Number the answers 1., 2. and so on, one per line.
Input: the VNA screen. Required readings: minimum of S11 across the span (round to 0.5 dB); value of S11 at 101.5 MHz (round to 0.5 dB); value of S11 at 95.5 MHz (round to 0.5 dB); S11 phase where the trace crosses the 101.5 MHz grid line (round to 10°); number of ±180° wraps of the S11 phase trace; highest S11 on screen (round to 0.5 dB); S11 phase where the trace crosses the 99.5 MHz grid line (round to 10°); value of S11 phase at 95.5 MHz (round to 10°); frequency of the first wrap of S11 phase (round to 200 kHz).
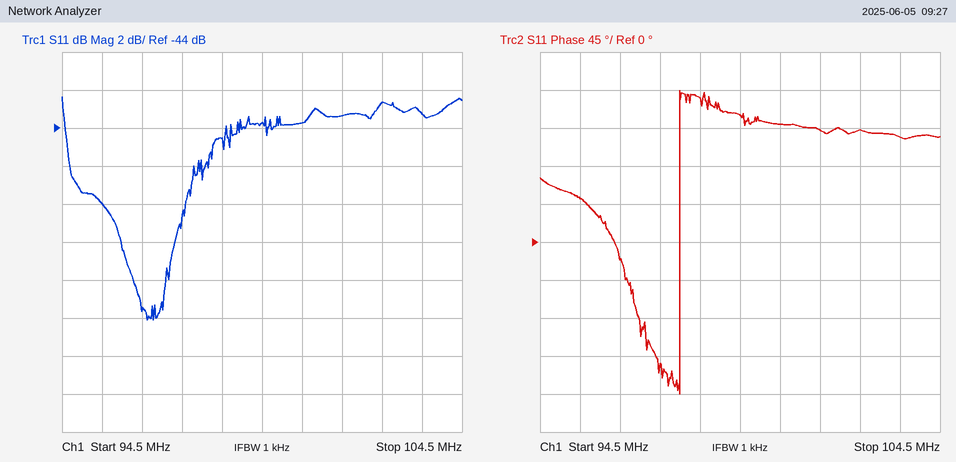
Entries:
1. -54.0 dB
2. -43.5 dB
3. -48.0 dB
4. 130°
5. 1
6. -42.5 dB
7. 150°
8. 50°
9. 98.0 MHz
